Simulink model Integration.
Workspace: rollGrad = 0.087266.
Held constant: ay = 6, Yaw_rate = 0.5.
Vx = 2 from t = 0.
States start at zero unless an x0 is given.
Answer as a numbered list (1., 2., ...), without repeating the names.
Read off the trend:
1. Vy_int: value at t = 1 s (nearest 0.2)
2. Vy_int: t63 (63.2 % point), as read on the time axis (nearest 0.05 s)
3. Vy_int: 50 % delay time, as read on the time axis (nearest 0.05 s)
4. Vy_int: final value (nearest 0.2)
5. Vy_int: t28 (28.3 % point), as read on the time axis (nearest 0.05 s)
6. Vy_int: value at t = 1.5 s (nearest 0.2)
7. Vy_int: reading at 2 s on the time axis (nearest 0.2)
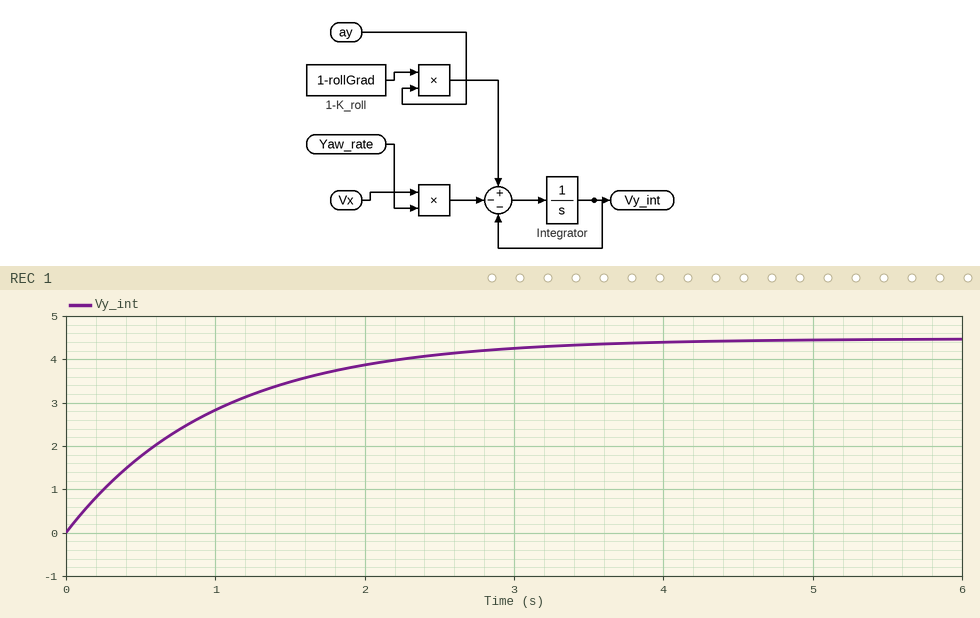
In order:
1. 2.8
2. 1.00 s
3. 0.70 s
4. 4.4
5. 0.35 s
6. 3.4
7. 3.8
